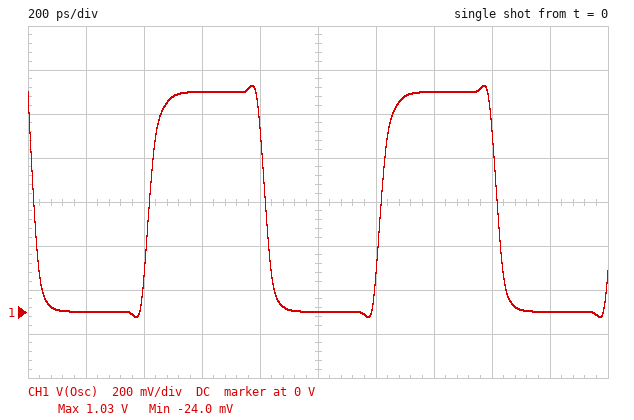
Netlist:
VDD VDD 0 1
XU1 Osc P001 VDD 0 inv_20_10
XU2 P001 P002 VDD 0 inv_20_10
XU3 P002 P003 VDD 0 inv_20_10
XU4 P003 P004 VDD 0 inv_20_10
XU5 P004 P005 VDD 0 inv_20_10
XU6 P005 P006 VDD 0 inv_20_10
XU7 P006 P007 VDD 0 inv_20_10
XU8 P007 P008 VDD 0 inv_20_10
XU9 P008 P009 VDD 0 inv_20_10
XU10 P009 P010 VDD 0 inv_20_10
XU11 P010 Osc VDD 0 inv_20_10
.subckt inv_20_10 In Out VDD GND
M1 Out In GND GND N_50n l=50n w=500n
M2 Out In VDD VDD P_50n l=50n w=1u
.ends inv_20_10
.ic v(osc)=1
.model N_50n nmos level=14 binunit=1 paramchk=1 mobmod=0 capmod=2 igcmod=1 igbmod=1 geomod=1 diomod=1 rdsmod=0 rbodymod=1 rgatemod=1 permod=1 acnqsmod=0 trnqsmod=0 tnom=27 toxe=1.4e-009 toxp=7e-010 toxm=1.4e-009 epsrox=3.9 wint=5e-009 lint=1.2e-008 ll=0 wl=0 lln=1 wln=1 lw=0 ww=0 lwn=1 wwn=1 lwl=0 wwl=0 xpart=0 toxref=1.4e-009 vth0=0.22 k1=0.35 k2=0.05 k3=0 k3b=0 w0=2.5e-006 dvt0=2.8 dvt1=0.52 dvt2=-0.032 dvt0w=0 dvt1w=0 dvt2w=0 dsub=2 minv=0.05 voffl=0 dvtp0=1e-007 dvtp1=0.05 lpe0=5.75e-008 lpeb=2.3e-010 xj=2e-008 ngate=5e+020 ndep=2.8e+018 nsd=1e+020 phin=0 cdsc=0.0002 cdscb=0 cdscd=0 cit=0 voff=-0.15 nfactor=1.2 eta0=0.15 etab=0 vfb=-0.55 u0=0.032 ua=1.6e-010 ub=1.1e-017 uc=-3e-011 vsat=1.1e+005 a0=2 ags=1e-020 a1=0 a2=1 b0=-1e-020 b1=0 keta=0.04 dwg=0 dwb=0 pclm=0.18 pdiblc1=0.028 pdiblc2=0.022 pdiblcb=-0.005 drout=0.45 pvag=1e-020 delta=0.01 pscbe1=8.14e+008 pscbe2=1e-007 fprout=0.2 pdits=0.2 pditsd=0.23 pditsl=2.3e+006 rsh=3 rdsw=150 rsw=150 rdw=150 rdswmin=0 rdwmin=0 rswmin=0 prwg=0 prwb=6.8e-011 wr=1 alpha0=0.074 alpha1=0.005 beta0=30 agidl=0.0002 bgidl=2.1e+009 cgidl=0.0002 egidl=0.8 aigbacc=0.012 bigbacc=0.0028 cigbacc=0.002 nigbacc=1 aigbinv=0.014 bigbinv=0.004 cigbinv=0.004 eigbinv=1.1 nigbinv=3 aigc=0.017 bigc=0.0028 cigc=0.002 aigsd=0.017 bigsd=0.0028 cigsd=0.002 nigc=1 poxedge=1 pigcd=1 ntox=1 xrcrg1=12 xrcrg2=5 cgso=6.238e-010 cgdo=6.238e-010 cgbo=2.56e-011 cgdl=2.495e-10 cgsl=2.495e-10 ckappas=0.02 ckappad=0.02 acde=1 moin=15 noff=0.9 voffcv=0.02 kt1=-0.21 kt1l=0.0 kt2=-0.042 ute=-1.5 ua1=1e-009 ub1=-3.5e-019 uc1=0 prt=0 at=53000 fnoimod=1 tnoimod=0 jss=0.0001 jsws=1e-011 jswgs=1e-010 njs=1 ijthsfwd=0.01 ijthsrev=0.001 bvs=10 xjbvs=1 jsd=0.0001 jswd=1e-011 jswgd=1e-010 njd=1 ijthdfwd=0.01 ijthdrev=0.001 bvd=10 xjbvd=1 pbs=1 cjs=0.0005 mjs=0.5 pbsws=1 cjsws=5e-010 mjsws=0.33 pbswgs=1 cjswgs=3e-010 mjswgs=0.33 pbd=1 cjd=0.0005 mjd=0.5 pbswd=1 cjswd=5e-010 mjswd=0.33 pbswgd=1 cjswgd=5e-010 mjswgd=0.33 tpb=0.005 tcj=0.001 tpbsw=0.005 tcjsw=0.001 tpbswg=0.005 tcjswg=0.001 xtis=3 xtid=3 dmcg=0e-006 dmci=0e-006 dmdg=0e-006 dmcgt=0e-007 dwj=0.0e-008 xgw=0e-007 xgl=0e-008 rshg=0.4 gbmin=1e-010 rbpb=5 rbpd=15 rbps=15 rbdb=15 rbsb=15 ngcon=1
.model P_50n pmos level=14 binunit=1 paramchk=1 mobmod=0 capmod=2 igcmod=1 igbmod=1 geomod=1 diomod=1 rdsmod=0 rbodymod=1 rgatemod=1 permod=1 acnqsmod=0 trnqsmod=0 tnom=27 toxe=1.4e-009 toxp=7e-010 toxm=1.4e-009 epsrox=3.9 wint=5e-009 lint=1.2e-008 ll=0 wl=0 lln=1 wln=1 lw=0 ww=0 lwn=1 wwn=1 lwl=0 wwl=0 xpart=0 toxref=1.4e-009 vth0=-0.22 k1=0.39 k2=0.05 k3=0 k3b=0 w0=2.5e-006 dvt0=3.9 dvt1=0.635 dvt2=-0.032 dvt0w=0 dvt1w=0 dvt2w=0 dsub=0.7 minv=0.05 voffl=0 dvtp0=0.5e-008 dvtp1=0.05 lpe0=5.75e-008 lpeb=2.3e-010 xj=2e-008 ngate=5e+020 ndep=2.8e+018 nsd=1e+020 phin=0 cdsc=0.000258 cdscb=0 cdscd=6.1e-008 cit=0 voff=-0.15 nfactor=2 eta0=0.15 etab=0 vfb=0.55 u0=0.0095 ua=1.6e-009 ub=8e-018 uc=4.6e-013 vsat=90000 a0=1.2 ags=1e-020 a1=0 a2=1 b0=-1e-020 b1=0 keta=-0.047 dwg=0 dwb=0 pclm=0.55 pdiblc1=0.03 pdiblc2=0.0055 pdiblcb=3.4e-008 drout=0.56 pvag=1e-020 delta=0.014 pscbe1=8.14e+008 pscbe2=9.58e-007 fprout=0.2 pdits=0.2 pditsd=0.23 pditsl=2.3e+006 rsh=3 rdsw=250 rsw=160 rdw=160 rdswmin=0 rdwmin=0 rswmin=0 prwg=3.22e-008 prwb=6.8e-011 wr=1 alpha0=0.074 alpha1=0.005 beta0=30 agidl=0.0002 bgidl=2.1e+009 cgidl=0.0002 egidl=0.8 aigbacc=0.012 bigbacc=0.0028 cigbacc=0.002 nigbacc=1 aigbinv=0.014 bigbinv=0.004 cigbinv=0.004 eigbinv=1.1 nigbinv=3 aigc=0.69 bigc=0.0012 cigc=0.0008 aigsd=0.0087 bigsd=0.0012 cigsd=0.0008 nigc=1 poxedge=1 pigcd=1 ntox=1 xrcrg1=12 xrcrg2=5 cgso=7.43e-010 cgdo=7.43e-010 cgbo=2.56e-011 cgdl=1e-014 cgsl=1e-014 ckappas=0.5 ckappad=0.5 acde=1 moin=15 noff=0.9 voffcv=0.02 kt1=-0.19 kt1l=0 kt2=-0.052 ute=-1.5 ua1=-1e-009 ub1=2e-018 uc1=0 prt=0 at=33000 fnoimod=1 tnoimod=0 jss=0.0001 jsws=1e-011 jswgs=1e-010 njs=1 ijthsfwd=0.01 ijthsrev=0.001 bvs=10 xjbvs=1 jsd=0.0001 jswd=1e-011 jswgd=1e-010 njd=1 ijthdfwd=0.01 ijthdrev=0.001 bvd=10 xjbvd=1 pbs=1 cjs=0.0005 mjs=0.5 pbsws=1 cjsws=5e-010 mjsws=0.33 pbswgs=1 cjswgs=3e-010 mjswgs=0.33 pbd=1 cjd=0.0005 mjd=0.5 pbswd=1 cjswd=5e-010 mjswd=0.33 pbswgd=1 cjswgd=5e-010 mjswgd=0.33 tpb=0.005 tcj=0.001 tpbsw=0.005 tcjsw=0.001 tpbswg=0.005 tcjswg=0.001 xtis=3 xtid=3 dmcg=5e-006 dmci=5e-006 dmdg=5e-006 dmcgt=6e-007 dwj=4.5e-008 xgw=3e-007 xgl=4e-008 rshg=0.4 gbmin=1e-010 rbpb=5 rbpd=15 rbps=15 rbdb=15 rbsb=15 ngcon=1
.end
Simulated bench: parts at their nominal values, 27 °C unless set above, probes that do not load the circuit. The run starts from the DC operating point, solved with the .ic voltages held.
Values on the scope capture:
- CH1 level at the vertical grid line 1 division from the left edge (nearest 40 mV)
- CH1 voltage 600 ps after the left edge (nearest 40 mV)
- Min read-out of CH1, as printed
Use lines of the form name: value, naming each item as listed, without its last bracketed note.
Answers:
CH1 level at the vertical grid line 1 division from the left edge: 0 V
CH1 voltage 600 ps after the left edge: 1.00 V
Min read-out of CH1, as printed: -24.0 mV
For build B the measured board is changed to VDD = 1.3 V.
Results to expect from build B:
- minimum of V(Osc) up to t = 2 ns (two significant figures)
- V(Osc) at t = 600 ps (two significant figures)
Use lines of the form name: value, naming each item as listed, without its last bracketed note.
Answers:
minimum of V(Osc) up to t = 2 ns: -26 mV
V(Osc) at t = 600 ps: 1.3 V
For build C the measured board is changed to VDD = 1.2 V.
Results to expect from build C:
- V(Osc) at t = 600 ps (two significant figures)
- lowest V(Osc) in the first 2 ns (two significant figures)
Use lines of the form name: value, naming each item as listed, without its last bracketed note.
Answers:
V(Osc) at t = 600 ps: 1.2 V
lowest V(Osc) in the first 2 ns: -25 mV
